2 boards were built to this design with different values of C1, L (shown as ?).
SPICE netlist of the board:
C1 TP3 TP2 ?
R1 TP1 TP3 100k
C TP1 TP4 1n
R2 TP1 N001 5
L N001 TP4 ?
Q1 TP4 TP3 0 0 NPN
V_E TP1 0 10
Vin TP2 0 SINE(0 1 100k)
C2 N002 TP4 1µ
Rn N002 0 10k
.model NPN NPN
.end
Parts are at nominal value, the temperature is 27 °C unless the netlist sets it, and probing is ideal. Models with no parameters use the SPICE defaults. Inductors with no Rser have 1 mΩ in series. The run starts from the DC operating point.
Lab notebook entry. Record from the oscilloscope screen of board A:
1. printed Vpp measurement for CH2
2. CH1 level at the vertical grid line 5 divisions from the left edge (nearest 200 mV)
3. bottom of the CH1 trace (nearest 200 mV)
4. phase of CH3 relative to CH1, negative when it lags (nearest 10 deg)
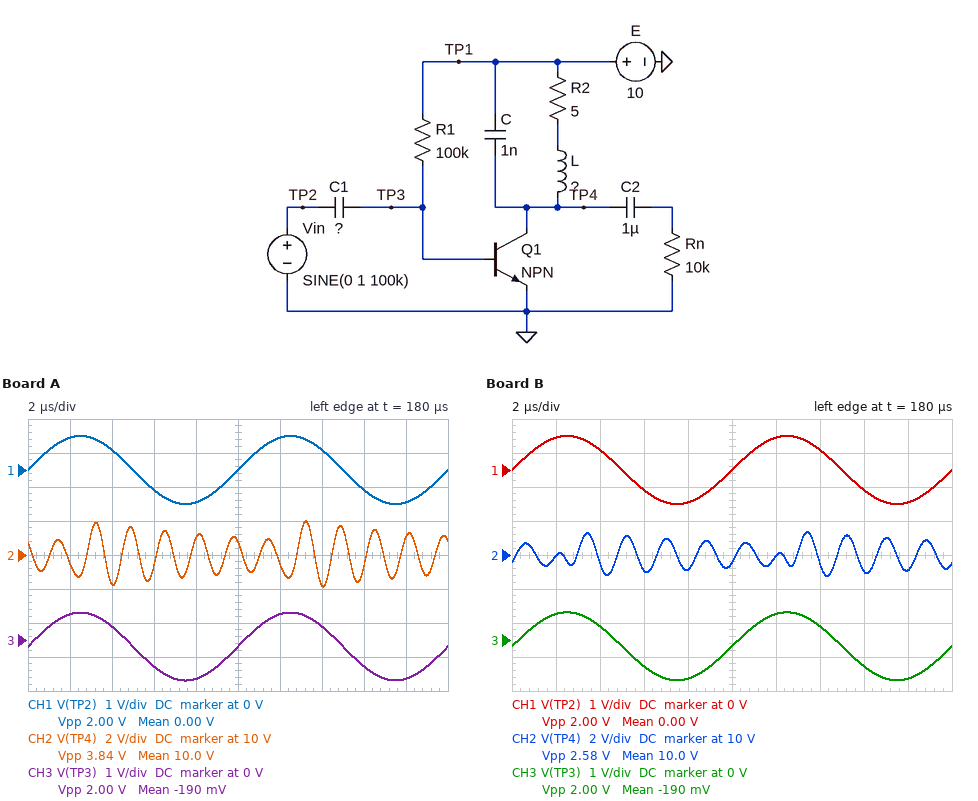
3.84 V
0 V
-1.0 V
0 deg
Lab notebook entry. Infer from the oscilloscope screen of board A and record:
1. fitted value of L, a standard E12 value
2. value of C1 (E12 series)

68 µH
820 nF
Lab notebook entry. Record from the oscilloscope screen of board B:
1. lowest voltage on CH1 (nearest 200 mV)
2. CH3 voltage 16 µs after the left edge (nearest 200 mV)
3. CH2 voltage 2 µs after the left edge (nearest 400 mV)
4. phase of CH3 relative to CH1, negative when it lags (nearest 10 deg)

-1.0 V
-800 mV
10.0 V
0 deg
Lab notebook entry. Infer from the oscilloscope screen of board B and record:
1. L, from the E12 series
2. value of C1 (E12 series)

82 µH
820 nF
